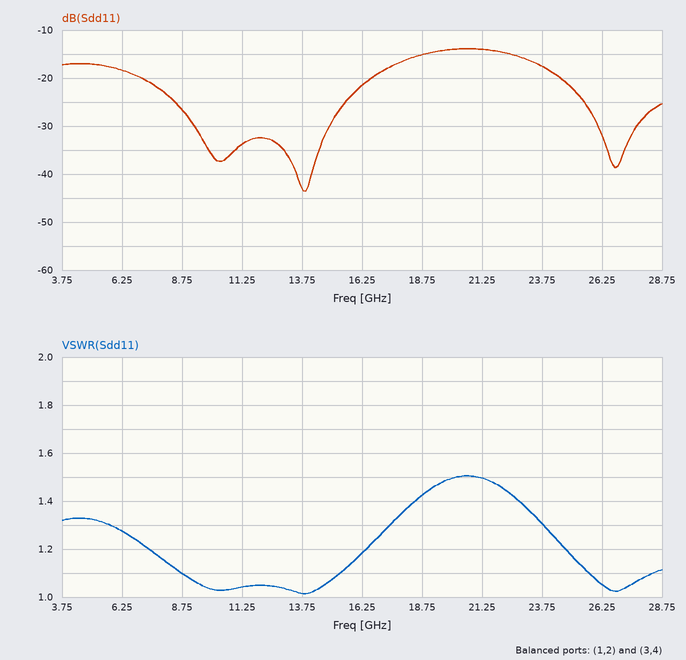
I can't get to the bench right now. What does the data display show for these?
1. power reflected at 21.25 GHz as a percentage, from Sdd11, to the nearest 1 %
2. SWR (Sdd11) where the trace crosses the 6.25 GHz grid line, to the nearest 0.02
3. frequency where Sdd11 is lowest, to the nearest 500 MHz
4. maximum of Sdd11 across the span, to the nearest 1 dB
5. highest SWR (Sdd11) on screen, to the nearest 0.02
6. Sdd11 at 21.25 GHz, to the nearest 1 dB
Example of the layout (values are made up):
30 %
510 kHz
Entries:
4 %
1.28
14.0 GHz
-14 dB
1.50
-14 dB
